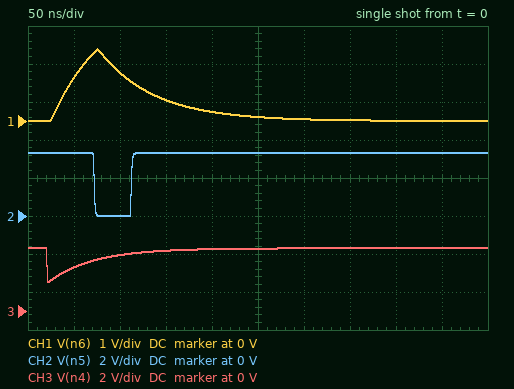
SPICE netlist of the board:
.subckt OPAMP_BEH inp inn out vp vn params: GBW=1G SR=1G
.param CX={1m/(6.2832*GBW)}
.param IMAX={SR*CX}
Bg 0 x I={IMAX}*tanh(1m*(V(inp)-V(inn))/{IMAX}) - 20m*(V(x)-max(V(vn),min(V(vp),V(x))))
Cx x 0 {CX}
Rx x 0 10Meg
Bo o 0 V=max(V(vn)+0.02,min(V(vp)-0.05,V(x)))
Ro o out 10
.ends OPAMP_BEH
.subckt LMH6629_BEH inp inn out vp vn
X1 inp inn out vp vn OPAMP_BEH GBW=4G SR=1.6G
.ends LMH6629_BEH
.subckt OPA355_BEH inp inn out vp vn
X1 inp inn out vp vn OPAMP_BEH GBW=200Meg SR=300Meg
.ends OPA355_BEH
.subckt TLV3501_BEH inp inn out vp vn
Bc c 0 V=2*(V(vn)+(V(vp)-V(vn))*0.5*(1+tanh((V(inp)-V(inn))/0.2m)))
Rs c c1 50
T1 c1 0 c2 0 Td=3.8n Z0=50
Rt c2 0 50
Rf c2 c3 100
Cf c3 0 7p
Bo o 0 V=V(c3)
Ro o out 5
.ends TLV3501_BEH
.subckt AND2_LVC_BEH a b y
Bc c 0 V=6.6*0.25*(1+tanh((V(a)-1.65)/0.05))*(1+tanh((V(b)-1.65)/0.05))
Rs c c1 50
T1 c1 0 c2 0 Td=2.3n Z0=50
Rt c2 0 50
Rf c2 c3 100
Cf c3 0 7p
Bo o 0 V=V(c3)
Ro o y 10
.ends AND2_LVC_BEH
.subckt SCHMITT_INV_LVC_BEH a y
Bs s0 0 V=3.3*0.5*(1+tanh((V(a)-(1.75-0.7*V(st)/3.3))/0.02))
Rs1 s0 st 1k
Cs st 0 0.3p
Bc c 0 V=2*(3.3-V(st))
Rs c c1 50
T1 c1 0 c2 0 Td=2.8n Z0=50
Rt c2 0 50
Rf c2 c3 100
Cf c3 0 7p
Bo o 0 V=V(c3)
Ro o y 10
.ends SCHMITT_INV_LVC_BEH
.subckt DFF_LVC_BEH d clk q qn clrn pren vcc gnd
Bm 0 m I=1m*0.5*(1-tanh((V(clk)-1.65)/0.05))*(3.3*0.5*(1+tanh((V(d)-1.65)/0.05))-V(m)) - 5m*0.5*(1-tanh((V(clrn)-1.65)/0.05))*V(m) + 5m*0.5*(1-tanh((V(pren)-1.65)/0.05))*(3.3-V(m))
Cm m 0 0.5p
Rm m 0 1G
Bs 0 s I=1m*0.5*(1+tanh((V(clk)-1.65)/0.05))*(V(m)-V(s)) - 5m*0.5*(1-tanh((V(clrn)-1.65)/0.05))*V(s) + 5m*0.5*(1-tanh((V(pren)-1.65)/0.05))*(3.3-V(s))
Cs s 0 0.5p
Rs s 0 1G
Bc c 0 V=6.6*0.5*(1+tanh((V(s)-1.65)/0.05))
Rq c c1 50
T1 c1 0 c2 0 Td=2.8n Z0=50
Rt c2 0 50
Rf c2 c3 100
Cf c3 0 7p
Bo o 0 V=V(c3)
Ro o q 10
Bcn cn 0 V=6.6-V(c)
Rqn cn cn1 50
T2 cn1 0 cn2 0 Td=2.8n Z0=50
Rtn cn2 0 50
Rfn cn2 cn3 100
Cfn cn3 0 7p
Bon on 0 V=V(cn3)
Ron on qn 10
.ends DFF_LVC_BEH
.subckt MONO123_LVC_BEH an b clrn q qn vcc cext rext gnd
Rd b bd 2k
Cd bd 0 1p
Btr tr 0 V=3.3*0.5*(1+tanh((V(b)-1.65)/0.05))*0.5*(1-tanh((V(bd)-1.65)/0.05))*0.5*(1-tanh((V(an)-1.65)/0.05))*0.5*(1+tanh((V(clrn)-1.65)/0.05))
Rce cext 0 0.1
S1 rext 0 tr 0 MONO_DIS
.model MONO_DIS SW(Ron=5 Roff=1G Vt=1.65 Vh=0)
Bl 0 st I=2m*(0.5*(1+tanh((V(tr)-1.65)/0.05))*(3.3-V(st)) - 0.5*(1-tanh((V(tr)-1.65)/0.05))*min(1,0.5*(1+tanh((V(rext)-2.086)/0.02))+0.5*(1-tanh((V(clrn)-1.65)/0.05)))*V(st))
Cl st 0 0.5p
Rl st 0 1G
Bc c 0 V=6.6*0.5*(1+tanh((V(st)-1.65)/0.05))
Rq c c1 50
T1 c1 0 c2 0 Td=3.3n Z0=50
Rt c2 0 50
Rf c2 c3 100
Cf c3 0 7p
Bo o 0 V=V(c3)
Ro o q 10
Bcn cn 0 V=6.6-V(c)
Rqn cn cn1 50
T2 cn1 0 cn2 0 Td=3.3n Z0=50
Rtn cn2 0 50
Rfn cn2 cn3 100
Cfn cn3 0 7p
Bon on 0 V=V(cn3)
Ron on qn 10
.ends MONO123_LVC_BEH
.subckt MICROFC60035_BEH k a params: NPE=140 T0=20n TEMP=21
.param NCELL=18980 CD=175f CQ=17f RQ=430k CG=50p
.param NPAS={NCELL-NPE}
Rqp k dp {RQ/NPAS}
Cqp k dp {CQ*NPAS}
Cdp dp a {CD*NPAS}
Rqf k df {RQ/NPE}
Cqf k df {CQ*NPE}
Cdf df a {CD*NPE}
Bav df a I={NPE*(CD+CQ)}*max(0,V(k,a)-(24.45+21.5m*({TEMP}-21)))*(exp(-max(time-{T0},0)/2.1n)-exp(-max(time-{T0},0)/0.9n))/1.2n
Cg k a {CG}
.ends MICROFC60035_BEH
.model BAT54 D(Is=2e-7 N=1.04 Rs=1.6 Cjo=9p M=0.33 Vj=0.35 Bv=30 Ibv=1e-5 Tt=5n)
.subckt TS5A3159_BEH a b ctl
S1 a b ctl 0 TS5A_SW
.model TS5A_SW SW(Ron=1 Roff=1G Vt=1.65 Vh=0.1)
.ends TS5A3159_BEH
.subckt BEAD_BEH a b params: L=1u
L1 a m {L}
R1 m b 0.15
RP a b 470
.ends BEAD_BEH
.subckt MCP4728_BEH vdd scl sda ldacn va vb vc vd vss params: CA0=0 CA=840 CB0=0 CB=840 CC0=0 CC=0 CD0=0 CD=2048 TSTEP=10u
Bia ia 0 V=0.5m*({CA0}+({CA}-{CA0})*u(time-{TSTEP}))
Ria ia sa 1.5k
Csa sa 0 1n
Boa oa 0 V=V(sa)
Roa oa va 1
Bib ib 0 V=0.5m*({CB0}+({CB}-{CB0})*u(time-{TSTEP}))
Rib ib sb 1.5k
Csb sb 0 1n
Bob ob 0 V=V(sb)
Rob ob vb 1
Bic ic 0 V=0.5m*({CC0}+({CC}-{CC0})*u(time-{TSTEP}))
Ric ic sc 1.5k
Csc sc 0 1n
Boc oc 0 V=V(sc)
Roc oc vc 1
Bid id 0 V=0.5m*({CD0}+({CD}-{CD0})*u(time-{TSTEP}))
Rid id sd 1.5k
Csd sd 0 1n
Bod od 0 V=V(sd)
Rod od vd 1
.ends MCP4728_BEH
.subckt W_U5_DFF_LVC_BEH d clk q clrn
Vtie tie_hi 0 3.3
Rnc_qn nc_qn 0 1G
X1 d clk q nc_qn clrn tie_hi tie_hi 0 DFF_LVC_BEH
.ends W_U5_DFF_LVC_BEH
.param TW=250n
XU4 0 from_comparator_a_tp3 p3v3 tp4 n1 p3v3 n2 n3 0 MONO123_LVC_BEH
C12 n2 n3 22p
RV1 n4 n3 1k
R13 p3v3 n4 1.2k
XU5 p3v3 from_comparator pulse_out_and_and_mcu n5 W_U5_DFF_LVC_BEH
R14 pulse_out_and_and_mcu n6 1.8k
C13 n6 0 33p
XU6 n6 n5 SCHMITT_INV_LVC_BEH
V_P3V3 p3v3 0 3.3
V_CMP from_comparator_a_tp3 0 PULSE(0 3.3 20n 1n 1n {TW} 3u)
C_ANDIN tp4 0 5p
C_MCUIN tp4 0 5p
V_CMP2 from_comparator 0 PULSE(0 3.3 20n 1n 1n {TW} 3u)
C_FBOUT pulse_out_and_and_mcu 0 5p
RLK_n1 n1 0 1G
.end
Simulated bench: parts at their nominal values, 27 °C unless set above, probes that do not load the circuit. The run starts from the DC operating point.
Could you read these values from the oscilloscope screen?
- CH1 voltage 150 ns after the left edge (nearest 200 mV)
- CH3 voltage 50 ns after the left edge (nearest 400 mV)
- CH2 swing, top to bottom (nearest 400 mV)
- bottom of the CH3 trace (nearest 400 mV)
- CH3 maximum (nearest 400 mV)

600 mV
2.4 V
3.2 V
1.6 V
3.2 V
